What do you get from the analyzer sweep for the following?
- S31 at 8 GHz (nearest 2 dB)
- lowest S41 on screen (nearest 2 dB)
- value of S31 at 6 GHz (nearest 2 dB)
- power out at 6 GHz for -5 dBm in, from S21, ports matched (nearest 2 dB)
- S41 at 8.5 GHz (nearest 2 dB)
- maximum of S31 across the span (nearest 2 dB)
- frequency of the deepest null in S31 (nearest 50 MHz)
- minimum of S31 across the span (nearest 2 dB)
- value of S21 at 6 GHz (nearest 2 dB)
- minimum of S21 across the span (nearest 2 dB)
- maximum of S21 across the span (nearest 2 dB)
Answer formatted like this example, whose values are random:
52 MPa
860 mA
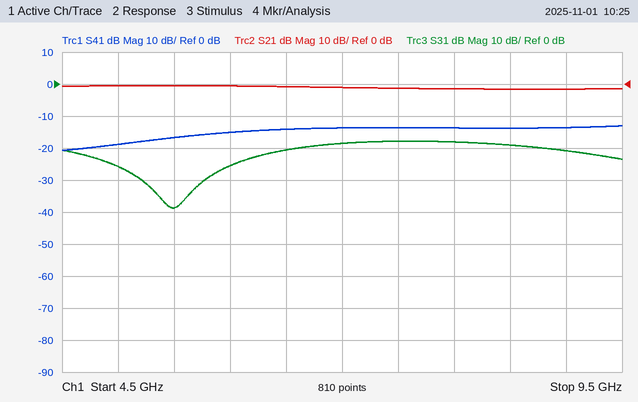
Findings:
-18 dB
-20 dB
-26 dB
-6 dBm
-14 dB
-18 dB
5.50 GHz
-38 dB
0 dB
-2 dB
0 dB
